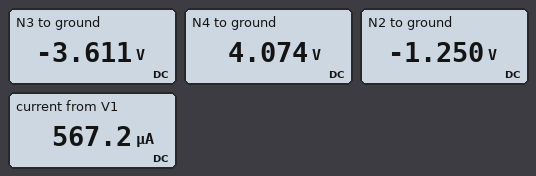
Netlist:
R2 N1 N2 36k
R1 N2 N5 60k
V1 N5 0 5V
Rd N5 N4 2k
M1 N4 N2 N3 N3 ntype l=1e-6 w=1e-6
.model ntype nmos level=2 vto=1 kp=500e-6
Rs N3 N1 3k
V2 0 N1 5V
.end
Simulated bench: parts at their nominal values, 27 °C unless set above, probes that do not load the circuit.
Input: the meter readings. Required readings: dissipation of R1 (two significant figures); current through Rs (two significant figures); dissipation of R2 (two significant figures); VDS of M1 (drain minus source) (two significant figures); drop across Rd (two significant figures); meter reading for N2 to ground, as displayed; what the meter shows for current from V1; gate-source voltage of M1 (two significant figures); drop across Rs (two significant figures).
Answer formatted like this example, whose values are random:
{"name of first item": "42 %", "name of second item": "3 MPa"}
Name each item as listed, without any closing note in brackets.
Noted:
{"dissipation of R1": "650 µW", "current through Rs": "460 µA", "dissipation of R2": "390 µW", "VDS of M1 (drain minus source)": "7.7 V", "drop across Rd": "930 mV", "meter reading for N2 to ground, as displayed": "-1.250 V", "what the meter shows for current from V1": "567.2 µA", "gate-source voltage of M1": "2.4 V", "drop across Rs": "1.4 V"}
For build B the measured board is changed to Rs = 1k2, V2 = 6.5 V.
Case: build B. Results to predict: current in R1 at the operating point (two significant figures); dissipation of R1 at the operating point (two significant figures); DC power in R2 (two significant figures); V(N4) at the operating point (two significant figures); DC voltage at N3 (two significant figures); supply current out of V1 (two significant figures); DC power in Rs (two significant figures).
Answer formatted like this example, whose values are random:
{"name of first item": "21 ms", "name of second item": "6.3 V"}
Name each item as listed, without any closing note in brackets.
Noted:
{"current in R1 at the operating point": "120 µA", "dissipation of R1 at the operating point": "860 µW", "DC power in R2": "520 µW", "V(N4) at the operating point": "2.9 V", "DC voltage at N3": "-5.2 V", "supply current out of V1": "1.2 mA", "DC power in Rs": "1.3 mW"}
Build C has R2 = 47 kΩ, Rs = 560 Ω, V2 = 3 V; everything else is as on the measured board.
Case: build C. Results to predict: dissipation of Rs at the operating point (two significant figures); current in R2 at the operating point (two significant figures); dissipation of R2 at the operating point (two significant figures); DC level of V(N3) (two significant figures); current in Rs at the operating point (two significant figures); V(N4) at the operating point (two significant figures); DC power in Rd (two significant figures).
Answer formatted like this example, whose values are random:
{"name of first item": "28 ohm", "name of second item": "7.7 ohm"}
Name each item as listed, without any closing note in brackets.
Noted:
{"dissipation of Rs at the operating point": "530 µW", "current in R2 at the operating point": "75 µA", "dissipation of R2 at the operating point": "260 µW", "DC level of V(N3)": "-2.5 V", "current in Rs at the operating point": "970 µA", "V(N4) at the operating point": "3.1 V", "DC power in Rd": "1.9 mW"}
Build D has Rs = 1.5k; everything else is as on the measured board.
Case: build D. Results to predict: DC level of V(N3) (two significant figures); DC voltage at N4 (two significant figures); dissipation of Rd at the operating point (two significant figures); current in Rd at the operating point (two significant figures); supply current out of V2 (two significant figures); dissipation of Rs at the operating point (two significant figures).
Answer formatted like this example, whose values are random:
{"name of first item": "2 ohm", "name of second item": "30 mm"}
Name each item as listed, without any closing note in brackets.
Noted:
{"DC level of V(N3)": "-3.9 V", "DC voltage at N4": "3.6 V", "dissipation of Rd at the operating point": "1.0 mW", "current in Rd at the operating point": "710 µA", "supply current out of V2": "810 µA", "dissipation of Rs at the operating point": "760 µW"}
